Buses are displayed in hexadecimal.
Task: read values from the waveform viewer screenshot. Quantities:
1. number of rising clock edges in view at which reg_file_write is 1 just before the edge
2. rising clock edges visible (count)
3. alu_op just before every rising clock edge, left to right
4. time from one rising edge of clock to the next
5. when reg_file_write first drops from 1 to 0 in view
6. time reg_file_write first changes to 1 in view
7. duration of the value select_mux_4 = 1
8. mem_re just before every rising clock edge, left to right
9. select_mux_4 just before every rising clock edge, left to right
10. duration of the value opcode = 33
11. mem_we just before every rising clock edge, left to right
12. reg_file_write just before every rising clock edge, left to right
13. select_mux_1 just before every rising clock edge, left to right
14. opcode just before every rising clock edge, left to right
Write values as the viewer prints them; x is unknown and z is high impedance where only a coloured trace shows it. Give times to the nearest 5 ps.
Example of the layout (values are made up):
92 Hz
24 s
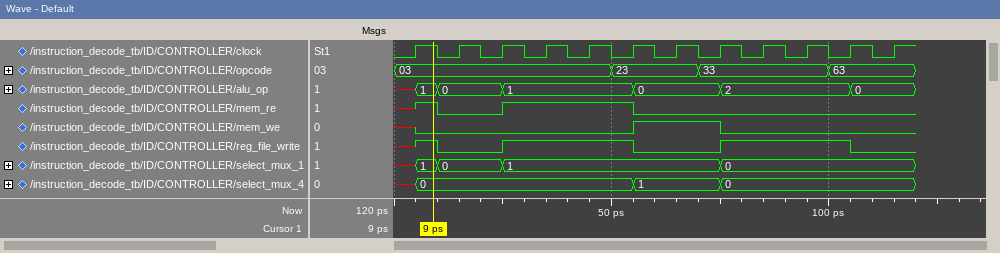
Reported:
6
12
x, 0, 0, 1, 1, 1, 0, 0, 2, 2, 2, 0
10 ps
10 ps
5 ps
20 ps
x 0 0 1 1 1 0 0 0 0 0 0
x, 0, 0, 0, 0, 0, 1, 1, 0, 0, 0, 0
30 ps
x 0 0 0 0 0 1 1 0 0 0 0
x 0 0 1 1 1 0 0 1 1 1 0
x, 0, 0, 1, 1, 1, 1, 1, 0, 0, 0, 0
03, 03, 03, 03, 03, 23, 23, 33, 33, 33, 63, 63
